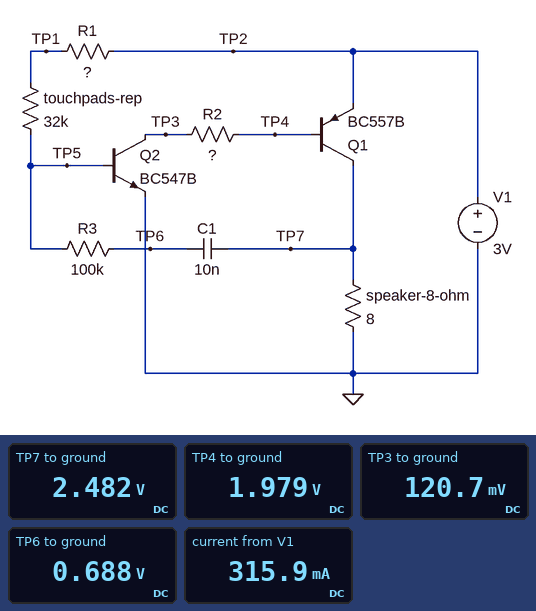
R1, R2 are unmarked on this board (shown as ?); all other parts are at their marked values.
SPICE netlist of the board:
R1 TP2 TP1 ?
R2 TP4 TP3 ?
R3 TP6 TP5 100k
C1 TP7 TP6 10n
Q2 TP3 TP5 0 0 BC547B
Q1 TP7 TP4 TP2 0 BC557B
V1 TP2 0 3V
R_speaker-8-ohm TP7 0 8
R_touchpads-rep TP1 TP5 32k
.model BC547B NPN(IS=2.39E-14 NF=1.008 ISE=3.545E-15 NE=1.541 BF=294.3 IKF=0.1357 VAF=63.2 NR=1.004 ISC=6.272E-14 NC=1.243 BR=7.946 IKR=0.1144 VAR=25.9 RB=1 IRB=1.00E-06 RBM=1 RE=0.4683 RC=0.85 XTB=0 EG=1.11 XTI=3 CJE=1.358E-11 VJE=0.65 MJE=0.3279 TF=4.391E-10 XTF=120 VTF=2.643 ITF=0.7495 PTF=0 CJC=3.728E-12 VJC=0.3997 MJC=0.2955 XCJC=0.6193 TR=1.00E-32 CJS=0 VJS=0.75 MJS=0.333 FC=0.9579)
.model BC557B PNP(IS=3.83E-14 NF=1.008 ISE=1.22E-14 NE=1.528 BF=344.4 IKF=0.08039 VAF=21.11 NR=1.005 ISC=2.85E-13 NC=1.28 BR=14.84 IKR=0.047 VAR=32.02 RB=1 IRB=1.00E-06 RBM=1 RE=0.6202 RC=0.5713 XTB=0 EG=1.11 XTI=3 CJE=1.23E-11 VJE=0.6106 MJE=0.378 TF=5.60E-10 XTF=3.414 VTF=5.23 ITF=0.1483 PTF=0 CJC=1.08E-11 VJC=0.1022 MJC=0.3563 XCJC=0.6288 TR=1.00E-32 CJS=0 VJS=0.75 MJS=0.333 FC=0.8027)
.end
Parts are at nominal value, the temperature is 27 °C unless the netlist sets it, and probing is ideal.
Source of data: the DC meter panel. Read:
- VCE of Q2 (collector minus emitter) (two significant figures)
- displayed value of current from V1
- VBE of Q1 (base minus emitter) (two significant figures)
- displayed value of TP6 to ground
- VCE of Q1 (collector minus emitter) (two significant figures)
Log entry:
120 mV
315.9 mA
-1.0 V
0.688 V
-520 mV
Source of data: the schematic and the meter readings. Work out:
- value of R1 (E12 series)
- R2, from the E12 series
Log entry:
33 kΩ
330 Ω
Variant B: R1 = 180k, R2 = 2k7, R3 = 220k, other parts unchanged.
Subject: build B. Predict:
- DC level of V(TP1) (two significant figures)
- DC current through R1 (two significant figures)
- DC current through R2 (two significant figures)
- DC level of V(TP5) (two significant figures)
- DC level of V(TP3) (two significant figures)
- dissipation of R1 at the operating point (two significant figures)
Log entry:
990 mV
11 µA
770 µA
630 mV
78 mV
22 µW
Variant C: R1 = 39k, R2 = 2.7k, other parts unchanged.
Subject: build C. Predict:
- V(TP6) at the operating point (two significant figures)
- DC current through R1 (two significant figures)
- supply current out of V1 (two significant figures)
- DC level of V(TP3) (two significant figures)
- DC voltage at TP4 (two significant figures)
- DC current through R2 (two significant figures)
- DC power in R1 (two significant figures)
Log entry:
640 mV
33 µA
120 mA
48 mV
2.2 V
780 µA
43 µW
